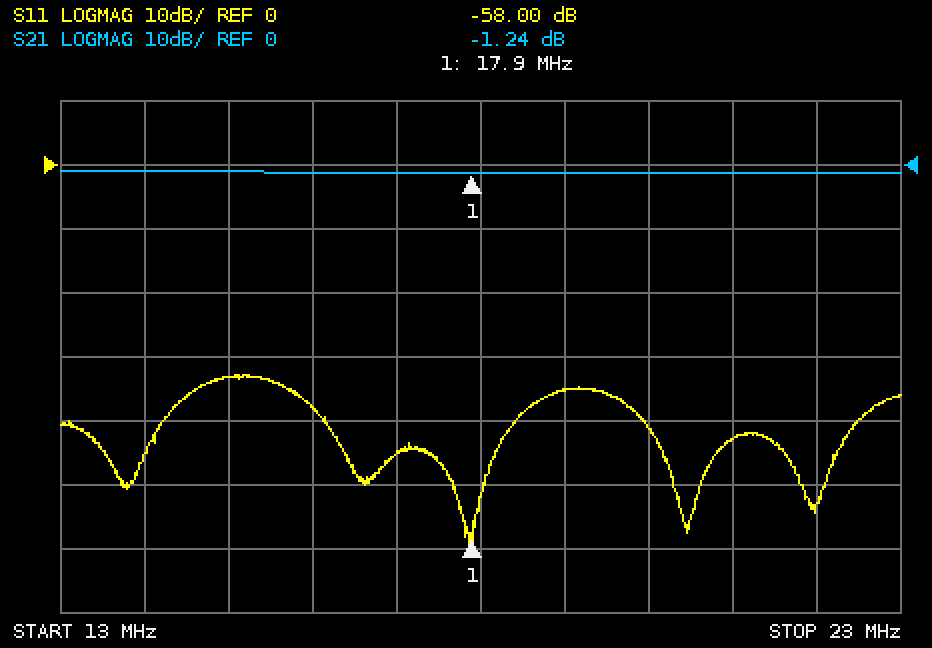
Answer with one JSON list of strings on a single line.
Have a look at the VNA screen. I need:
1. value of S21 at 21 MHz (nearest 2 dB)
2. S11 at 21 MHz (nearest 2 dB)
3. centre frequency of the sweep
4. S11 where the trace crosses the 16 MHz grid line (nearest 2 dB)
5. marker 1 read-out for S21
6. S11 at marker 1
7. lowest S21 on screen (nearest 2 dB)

["-2 dB", "-42 dB", "18 MHz", "-38 dB", "-1.24 dB", "-58.00 dB", "-2 dB"]
